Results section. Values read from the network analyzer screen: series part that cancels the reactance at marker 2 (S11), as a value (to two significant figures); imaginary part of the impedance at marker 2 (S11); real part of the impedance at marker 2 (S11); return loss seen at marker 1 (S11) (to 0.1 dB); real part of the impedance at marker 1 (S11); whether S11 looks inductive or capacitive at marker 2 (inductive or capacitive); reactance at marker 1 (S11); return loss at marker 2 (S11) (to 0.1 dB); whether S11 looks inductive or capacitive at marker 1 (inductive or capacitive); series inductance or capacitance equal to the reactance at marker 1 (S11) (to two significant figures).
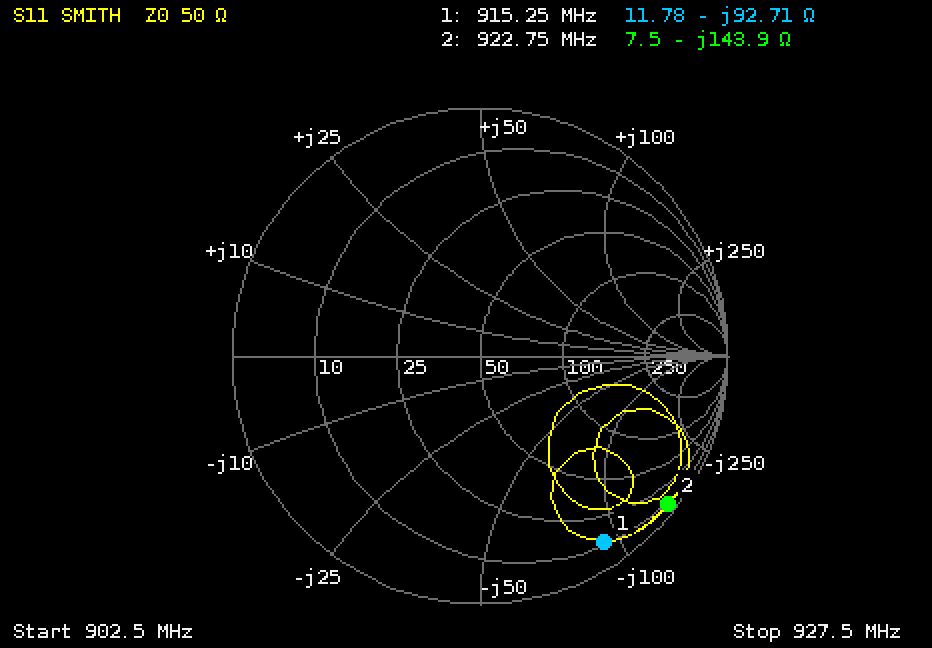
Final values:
25 nH
-143.9 Ω
7.5 Ω
0.9 dB
11.78 Ω
capacitive
-92.71 Ω
0.3 dB
capacitive
1.9 pF
